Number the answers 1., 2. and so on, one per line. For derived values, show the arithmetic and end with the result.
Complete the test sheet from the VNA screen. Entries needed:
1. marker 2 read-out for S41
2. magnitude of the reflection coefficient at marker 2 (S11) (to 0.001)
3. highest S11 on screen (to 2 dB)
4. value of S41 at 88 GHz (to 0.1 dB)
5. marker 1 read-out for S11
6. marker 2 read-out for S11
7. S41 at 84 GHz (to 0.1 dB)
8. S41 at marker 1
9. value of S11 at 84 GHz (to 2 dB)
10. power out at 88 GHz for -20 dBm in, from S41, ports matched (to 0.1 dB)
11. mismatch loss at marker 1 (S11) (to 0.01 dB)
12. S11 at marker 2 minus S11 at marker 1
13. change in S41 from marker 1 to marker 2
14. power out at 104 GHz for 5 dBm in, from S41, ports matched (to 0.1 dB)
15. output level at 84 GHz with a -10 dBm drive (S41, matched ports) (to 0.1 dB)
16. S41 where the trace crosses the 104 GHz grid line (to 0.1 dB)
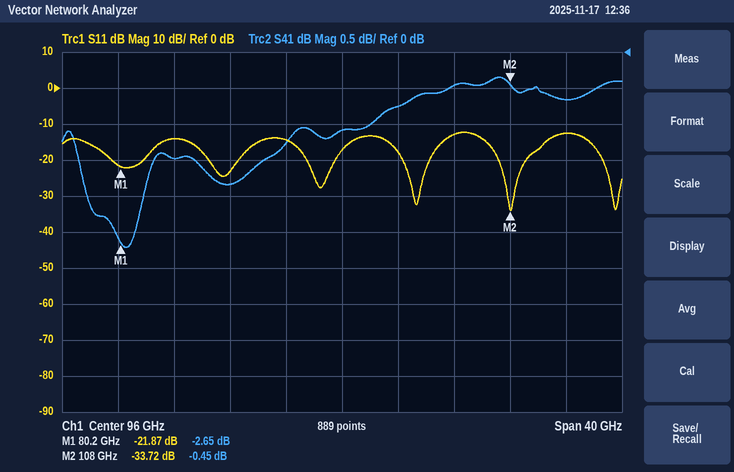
1. -0.45 dB
2. 10^(-33.72/20) ≈ 0.021
3. -12 dB
4. -1.8 dB
5. -21.87 dB
6. -33.72 dB
7. -1.5 dB
8. -2.65 dB
9. -14 dB
10. -20 dBm + (-1.8 dB) = -21.8 dBm
11. −10 log10(1 − 10^(-21.87/10)) ≈ 0.03 dB
12. -33.72 − (-21.87) = -11.85 dB
13. -0.45 − (-2.65) = 2.20 dB
14. 5 dBm + (-0.5 dB) = 4.5 dBm
15. -10 dBm + (-1.5 dB) = -11.5 dBm
16. -0.5 dB
